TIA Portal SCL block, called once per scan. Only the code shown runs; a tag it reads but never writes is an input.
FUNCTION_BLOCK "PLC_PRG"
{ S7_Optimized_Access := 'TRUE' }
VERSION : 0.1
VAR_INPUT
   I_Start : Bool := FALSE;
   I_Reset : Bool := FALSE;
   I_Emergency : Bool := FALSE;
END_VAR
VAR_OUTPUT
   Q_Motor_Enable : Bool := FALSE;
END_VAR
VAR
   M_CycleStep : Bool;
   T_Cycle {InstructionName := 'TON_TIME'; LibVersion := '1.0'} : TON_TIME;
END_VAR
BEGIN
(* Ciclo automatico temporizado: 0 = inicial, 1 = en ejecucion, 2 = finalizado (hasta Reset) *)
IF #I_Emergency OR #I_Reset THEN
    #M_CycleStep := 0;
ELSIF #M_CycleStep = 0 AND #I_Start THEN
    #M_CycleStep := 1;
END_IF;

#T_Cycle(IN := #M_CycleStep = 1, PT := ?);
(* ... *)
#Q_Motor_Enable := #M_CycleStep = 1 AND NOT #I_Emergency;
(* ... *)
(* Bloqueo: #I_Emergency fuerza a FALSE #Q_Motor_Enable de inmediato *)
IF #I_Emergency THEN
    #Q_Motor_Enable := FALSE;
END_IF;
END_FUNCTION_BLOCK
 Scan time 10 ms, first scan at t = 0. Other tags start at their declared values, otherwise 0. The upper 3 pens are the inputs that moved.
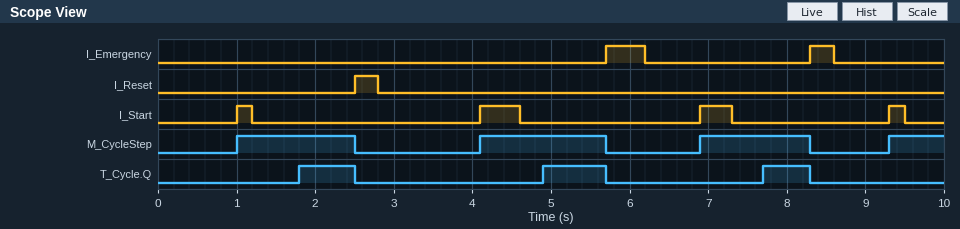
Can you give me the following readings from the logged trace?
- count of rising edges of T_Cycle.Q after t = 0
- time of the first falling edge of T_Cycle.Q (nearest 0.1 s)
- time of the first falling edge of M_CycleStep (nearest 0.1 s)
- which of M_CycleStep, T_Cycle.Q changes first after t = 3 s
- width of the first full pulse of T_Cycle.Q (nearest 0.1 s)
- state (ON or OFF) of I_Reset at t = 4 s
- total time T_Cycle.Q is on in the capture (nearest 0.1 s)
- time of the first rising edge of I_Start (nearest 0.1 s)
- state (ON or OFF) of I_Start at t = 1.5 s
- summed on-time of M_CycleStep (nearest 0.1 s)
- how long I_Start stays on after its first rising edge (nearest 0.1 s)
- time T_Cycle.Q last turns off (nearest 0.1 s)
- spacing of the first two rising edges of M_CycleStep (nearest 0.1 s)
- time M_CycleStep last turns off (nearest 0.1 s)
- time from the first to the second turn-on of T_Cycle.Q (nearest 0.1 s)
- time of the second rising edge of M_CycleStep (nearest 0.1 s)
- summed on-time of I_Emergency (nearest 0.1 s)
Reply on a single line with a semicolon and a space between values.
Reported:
3; 2.5 s; 2.5 s; M_CycleStep; 0.7 s; OFF; 2.1 s; 1.0 s; OFF; 5.2 s; 0.2 s; 8.3 s; 3.1 s; 8.3 s; 3.1 s; 4.1 s; 0.8 s
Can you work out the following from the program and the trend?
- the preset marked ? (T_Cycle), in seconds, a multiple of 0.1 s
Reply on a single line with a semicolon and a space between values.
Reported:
0.8 s
